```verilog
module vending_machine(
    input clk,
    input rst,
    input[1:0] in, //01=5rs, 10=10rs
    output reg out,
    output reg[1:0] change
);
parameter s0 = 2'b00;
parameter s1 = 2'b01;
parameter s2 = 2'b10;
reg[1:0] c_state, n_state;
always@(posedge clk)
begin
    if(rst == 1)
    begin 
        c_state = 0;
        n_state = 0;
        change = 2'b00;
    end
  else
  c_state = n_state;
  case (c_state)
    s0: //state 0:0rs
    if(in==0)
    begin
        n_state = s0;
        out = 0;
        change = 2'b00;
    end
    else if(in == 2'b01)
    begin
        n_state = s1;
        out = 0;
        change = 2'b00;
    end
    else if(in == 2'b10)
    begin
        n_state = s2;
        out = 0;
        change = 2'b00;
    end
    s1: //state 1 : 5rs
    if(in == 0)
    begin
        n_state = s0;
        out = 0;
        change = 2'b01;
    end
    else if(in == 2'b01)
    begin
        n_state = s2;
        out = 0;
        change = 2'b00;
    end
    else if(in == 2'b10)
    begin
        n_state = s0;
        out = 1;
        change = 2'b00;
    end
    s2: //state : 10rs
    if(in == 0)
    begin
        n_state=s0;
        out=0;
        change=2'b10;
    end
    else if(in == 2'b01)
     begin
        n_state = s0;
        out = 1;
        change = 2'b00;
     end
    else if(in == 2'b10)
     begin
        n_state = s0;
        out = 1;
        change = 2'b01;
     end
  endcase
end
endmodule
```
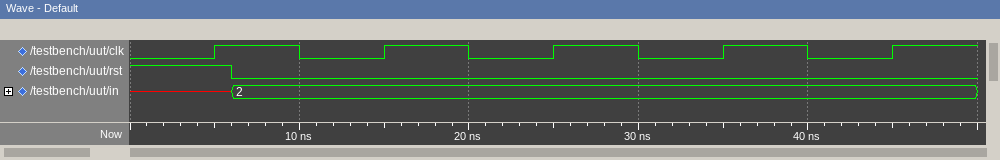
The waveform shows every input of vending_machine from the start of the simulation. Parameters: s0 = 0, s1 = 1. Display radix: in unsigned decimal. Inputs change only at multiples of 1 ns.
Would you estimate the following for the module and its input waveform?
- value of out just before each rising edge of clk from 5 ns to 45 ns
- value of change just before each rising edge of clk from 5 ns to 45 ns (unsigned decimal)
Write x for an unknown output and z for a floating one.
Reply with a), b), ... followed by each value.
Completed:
a) x x 0 1 0
b) x, 0, 0, 1, 0
